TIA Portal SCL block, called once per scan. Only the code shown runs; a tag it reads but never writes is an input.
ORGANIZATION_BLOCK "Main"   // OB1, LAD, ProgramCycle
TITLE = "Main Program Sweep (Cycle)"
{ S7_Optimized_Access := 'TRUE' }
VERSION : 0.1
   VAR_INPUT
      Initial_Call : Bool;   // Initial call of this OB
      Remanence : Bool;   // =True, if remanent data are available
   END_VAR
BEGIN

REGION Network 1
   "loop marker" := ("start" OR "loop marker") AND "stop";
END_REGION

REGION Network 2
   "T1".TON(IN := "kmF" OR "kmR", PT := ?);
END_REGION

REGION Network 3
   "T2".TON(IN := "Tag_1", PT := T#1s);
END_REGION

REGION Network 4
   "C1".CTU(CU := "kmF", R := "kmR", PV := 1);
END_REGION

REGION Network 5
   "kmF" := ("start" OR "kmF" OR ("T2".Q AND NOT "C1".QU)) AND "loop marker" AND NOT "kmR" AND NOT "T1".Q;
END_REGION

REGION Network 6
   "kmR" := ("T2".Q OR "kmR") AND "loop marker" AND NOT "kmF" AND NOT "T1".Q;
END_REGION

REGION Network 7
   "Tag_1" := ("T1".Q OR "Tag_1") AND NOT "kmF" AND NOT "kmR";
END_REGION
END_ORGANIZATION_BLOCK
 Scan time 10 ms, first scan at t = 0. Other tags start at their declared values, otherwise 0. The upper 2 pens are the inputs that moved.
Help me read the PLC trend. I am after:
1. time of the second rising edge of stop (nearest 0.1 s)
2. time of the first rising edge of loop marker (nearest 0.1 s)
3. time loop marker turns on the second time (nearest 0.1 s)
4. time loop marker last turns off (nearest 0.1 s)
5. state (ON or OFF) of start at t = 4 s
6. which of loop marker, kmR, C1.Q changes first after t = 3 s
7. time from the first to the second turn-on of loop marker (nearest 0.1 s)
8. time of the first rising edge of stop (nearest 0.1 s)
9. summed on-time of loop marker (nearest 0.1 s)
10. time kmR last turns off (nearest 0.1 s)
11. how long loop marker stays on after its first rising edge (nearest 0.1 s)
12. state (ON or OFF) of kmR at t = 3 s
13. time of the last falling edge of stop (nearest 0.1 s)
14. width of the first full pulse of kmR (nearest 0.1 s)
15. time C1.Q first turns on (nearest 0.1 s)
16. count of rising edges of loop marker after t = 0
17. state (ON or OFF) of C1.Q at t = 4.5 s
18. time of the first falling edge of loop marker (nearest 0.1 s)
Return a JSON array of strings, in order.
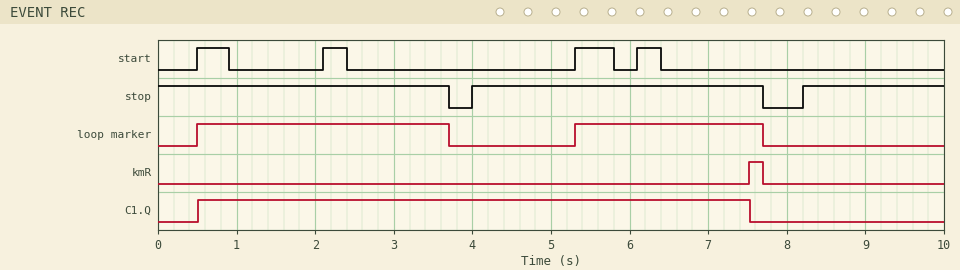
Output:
["8.2 s", "0.5 s", "5.3 s", "7.7 s", "OFF", "loop marker", "4.8 s", "4.0 s", "5.6 s", "7.7 s", "3.2 s", "OFF", "7.7 s", "0.2 s", "0.5 s", "2", "ON", "3.7 s"]
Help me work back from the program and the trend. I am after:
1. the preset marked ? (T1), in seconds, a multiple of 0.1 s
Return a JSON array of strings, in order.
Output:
["1.2 s"]
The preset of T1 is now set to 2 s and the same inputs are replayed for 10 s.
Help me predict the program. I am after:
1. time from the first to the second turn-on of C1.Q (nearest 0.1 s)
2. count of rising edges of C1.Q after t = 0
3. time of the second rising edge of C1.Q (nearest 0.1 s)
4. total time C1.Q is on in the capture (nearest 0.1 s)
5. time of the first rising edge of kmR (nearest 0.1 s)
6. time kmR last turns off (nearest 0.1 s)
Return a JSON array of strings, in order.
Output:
["4.8 s", "2", "5.3 s", "7.7 s", "3.5 s", "3.7 s"]
